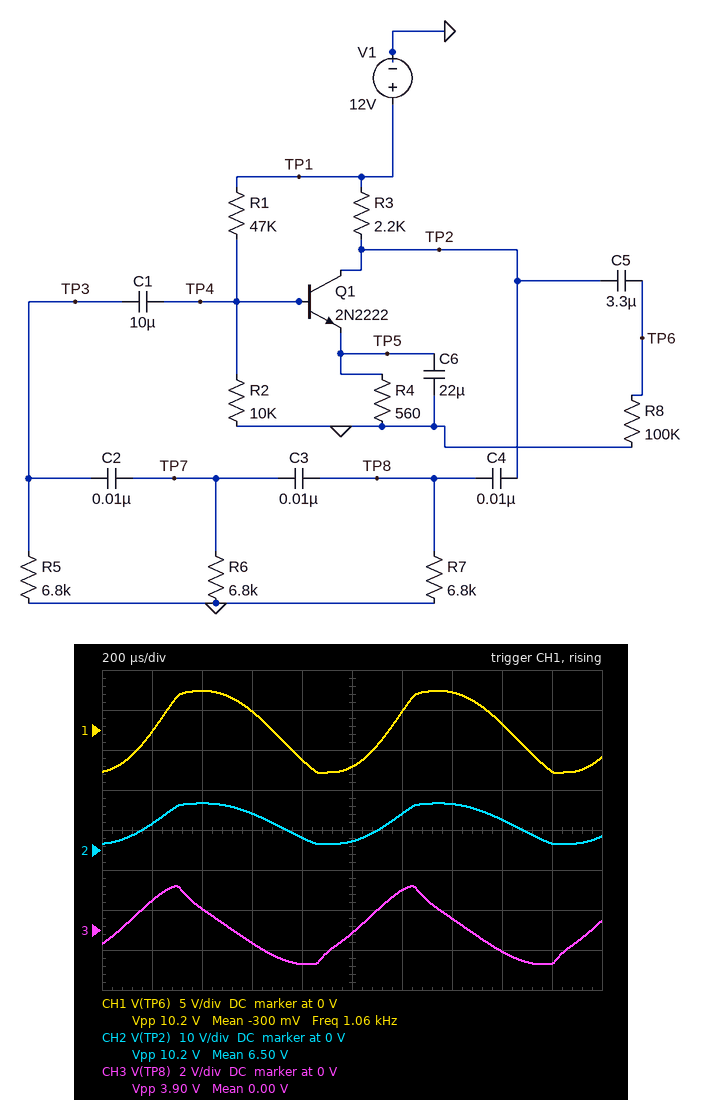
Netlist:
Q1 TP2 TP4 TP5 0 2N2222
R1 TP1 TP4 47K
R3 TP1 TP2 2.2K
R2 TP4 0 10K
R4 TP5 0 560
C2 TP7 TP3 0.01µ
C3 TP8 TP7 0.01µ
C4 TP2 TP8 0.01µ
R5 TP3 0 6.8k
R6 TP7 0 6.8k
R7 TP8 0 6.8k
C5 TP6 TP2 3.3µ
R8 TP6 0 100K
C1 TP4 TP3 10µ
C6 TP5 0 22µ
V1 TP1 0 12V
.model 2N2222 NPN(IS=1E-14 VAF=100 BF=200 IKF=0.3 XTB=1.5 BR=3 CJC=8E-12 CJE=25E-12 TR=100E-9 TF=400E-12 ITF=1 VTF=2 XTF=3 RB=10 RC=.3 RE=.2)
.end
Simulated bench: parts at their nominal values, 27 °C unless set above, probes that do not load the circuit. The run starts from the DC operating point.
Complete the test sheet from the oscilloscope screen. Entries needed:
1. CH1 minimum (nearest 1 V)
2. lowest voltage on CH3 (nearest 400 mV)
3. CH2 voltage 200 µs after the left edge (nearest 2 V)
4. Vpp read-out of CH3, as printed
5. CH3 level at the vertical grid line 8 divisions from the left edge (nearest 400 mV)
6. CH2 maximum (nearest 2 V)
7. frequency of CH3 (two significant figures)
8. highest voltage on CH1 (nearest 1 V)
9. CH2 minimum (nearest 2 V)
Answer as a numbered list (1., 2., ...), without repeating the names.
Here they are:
1. -5 V
2. -1.6 V
3. 6 V
4. 3.90 V
5. -1.2 V
6. 12 V
7. 1.1 kHz
8. 5 V
9. 2 V
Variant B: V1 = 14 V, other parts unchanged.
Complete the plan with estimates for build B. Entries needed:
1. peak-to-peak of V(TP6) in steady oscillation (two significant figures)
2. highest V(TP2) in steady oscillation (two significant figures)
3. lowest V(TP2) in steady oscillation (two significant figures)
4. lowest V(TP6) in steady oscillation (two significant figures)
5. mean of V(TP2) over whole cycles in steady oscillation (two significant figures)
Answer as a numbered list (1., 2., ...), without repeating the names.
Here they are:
1. 12 V
2. 14 V
3. 1.7 V
4. -5.8 V
5. 7.6 V
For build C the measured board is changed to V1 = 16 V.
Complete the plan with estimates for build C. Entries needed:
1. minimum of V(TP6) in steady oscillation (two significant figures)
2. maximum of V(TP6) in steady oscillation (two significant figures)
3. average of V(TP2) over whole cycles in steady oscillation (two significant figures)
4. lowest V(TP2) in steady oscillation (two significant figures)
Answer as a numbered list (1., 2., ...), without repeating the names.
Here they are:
1. -6.3 V
2. 7.2 V
3. 8.4 V
4. 2.0 V
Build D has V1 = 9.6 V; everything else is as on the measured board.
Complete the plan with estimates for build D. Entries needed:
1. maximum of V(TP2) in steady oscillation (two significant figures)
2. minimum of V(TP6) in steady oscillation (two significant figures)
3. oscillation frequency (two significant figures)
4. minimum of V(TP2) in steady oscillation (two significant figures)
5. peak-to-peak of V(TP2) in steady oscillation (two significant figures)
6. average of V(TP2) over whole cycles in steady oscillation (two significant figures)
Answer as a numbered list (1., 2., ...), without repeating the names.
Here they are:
1. 9.3 V
2. -3.7 V
3. 1.0 kHz
4. 2.2 V
5. 7.1 V
6. 5.8 V
